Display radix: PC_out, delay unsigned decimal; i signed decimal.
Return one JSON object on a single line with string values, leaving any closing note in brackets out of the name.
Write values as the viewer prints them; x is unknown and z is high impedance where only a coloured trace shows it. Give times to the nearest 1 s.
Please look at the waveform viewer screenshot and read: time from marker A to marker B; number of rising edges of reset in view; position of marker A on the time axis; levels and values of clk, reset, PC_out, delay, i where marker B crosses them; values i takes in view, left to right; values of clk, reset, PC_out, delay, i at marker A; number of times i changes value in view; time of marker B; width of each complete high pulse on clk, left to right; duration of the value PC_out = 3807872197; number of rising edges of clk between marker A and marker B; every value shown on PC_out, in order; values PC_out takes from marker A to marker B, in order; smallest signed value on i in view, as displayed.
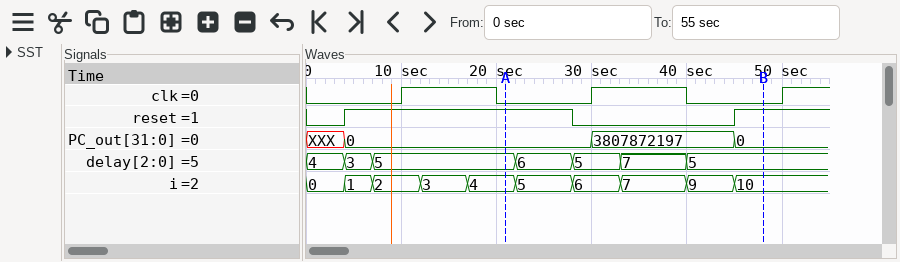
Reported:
{"time from marker A to marker B": "27 s", "number of rising edges of reset in view": "2", "position of marker A on the time axis": "21 s", "levels and values of clk, reset, PC_out, delay, i where marker B crosses them": "clk=0, reset=1, PC_out=0, delay=5, i=10", "values i takes in view, left to right": "0, 1, 2, 3, 4, 5, 6, 7, 9, 10", "values of clk, reset, PC_out, delay, i at marker A": "clk=0, reset=1, PC_out=0, delay=5, i=4", "number of times i changes value in view": "9", "time of marker B": "48 s", "width of each complete high pulse on clk, left to right": "10 s, 10 s", "duration of the value PC_out = 3807872197": "15 s", "number of rising edges of clk between marker A and marker B": "1", "every value shown on PC_out, in order": "XXX, 0, 3807872197, 0", "values PC_out takes from marker A to marker B, in order": "0, 3807872197, 0", "smallest signed value on i in view, as displayed": "0"}
